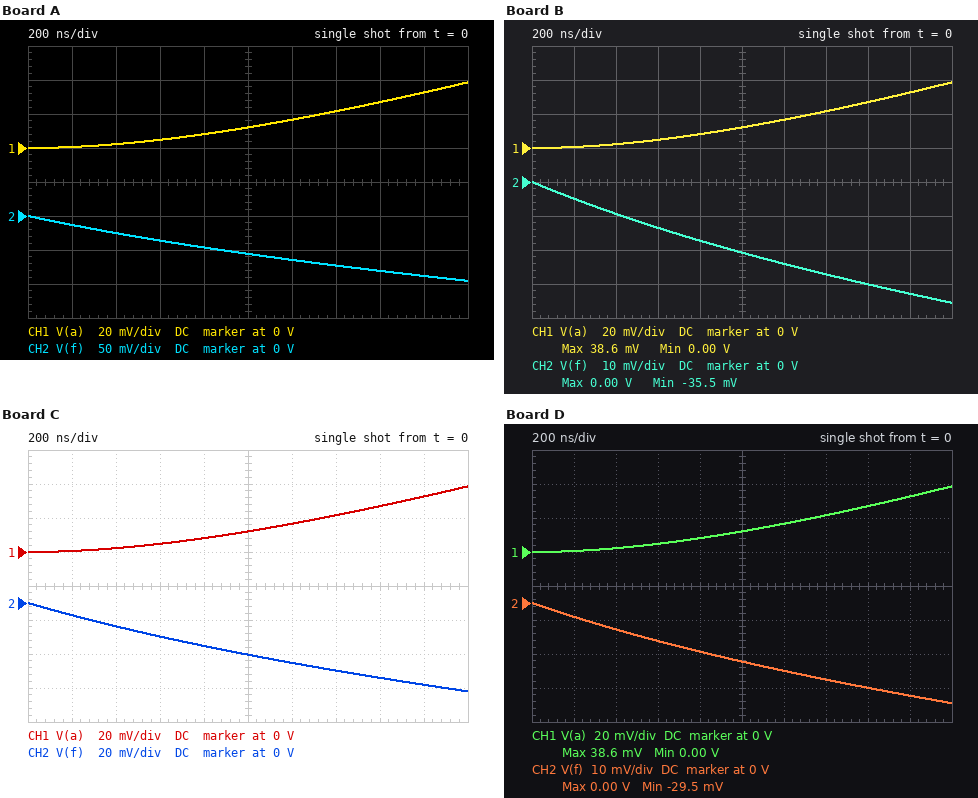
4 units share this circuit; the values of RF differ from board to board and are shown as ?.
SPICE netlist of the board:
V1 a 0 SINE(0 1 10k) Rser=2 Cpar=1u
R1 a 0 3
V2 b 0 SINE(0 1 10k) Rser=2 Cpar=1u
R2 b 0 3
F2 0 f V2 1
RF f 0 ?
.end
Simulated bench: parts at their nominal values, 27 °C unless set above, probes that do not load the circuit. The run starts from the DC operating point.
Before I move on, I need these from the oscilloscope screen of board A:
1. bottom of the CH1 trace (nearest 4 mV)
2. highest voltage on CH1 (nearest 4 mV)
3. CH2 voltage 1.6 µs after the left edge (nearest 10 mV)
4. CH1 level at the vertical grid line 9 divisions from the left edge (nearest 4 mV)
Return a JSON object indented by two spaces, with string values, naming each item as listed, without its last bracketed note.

{
  "bottom of the CH1 trace": "0 V",
  "highest voltage on CH1": "40 mV",
  "CH2 voltage 1.6 µs after the left edge": "-80 mV",
  "CH1 level at the vertical grid line 9 divisions from the left edge": "32 mV"
}
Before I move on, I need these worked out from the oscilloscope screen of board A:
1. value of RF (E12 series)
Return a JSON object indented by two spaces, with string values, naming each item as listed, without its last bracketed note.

{
  "value of RF": "2.2 Ω"
}
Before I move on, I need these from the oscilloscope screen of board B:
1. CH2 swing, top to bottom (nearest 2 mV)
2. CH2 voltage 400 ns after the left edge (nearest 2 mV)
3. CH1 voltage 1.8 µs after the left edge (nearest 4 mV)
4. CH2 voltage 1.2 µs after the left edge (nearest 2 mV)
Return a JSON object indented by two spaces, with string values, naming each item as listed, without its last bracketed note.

{
  "CH2 swing, top to bottom": "36 mV",
  "CH2 voltage 400 ns after the left edge": "-10 mV",
  "CH1 voltage 1.8 µs after the left edge": "32 mV",
  "CH2 voltage 1.2 µs after the left edge": "-24 mV"
}
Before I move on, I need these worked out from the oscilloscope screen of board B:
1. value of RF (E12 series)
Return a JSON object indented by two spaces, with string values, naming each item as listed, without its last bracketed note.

{
  "value of RF": "0.82 Ω"
}
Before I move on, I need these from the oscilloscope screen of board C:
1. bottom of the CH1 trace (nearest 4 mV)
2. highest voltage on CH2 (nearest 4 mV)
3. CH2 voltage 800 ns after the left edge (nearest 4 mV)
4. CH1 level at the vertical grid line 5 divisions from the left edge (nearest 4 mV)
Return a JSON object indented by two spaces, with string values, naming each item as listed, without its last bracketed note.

{
  "bottom of the CH1 trace": "0 V",
  "highest voltage on CH2": "0 V",
  "CH2 voltage 800 ns after the left edge": "-24 mV",
  "CH1 level at the vertical grid line 5 divisions from the left edge": "12 mV"
}
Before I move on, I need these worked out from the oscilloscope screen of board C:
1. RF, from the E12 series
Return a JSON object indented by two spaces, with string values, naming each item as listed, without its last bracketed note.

{
  "RF, from the E12 series": "1.2 Ω"
}
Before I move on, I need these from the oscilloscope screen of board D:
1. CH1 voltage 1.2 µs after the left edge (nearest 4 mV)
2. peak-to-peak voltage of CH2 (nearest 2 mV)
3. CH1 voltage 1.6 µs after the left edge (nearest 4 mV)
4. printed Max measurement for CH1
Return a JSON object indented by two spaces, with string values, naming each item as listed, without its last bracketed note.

{
  "CH1 voltage 1.2 µs after the left edge": "16 mV",
  "peak-to-peak voltage of CH2": "30 mV",
  "CH1 voltage 1.6 µs after the left edge": "28 mV",
  "printed Max measurement for CH1": "38.6 mV"
}
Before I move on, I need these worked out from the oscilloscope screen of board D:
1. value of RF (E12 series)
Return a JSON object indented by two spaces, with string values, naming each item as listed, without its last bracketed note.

{
  "value of RF": "0.68 Ω"
}
